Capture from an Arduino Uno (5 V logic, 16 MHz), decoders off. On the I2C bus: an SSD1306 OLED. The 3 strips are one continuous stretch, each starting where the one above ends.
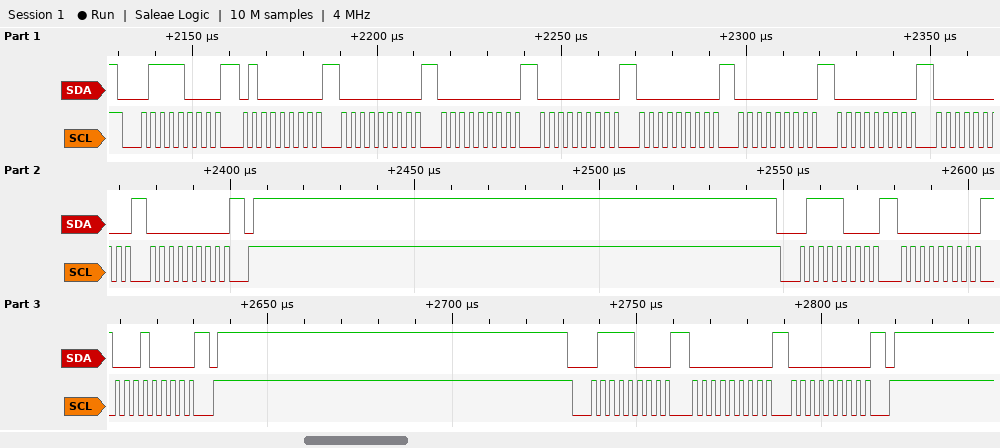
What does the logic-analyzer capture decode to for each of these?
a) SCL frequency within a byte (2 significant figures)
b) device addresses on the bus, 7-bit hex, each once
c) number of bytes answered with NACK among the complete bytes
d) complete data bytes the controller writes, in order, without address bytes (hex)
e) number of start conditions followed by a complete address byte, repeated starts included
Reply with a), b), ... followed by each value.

a) 400 kHz
b) 0x3C
c) 0
d) 40 00 00 00 00 00 00 00 00 00 10 00 00
e) 3
